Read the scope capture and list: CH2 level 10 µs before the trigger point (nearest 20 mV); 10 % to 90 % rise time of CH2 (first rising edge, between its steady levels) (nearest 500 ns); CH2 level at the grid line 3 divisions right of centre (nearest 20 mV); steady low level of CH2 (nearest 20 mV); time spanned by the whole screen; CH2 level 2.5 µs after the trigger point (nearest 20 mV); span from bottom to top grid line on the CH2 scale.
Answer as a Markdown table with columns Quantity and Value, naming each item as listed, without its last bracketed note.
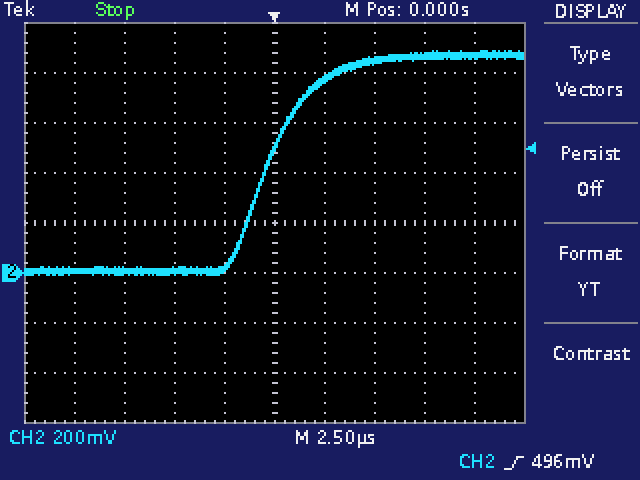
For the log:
| Quantity | Value |
|---|---|
| CH2 level 10 µs before the trigger point | 0 mV |
| 10 % to 90 % rise time of CH2 (first rising edge, between its steady levels) | 4.5 µs |
| CH2 level at the grid line 3 divisions right of centre | 860 mV |
| steady low level of CH2 | 0 mV |
| time spanned by the whole screen | 25 µs |
| CH2 level 2.5 µs after the trigger point | 780 mV |
| span from bottom to top grid line on the CH2 scale | 1.6 V |
